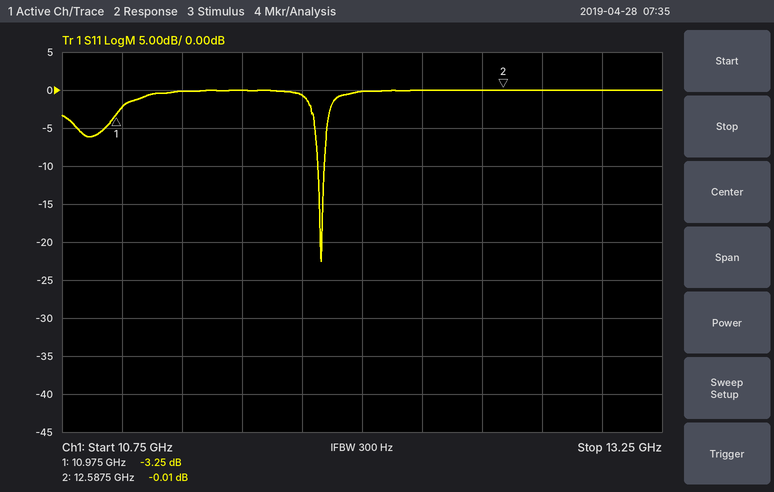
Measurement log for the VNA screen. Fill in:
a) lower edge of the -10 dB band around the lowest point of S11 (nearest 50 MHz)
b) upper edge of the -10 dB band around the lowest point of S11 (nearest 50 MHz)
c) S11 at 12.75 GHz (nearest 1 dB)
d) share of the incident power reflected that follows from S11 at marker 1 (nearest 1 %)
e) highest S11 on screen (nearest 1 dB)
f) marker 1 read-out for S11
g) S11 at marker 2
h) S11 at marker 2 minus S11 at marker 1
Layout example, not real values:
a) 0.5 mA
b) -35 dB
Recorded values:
a) 11.80 GHz
b) 11.85 GHz
c) 0 dB
d) 47 %
e) 0 dB
f) -3.25 dB
g) -0.01 dB
h) 3.24 dB
